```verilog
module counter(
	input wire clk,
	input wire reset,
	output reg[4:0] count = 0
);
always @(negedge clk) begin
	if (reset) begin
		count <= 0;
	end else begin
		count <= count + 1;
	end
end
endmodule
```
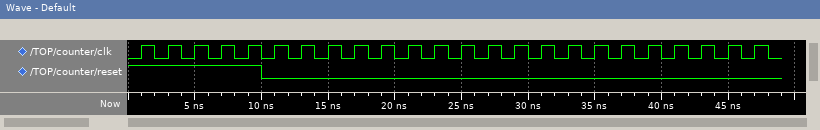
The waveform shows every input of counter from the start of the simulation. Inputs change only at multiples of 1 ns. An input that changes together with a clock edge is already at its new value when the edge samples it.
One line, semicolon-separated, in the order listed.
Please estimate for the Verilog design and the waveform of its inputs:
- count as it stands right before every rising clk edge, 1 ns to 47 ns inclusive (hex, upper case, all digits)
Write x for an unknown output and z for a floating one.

00, 00, 00, 00, 00, 01, 02, 03, 04, 05, 06, 07, 08, 09, 0A, 0B, 0C, 0D, 0E, 0F, 10, 11, 12, 13
